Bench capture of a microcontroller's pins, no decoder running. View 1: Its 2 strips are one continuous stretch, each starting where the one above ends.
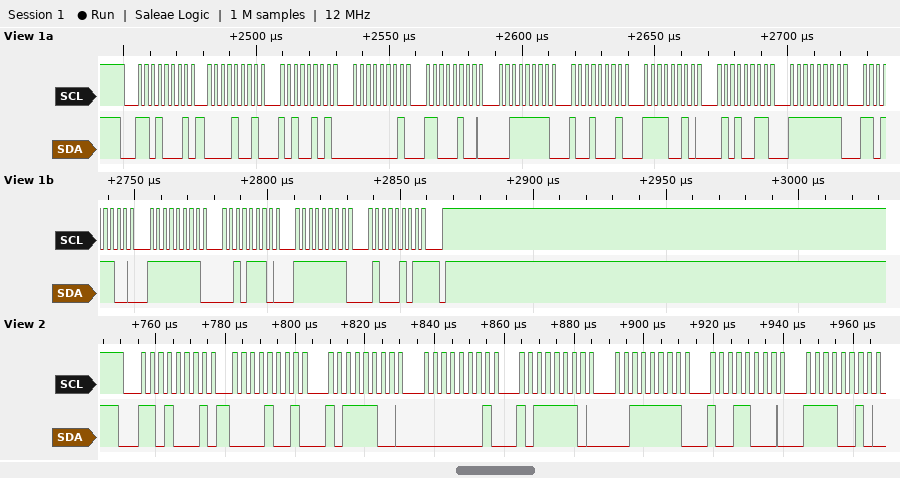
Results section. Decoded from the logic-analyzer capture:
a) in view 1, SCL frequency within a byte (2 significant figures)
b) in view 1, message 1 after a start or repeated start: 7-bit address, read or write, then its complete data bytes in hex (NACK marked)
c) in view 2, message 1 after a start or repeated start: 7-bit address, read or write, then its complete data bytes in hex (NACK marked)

400 kHz
0x68 read: 09 A5 01 C4 3F 91 F2 53 FF DC FF 2E FF 45 NACK
0x68 read: 09 BC 01 BE 3F 98 F2
